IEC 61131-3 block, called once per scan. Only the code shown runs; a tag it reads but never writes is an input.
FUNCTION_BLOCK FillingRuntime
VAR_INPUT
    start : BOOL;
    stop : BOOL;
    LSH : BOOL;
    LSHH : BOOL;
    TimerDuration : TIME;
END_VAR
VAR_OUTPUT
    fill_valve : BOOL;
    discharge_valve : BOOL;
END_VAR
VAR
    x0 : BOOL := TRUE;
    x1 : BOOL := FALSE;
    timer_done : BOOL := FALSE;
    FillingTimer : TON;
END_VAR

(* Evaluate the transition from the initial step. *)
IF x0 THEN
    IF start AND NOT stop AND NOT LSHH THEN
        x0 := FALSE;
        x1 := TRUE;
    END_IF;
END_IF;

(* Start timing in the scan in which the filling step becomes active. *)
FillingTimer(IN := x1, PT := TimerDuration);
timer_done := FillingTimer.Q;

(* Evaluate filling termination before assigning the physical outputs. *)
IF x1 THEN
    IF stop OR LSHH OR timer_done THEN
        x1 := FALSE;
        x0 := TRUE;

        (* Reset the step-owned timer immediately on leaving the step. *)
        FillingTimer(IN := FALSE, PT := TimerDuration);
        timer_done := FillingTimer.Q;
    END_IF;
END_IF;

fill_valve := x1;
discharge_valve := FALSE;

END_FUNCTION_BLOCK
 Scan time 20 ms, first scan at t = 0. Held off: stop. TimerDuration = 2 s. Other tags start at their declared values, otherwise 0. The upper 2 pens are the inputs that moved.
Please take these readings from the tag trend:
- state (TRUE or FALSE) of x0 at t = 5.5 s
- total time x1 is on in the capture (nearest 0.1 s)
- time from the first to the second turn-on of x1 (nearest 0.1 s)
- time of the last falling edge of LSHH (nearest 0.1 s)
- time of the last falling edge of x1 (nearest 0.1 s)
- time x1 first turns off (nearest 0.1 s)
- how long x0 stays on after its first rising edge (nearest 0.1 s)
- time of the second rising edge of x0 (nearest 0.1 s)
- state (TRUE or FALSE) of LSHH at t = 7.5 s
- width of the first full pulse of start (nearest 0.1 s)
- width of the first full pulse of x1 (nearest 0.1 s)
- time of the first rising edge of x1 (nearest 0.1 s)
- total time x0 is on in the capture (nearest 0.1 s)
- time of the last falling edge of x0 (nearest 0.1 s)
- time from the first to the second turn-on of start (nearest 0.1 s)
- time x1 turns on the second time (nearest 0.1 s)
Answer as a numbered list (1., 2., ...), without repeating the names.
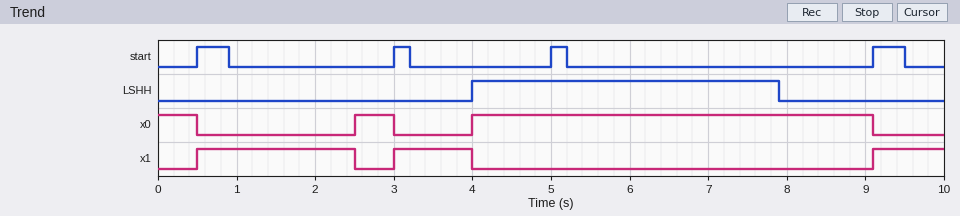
1. TRUE
2. 3.9 s
3. 2.5 s
4. 7.9 s
5. 4.0 s
6. 2.5 s
7. 0.5 s
8. 4.0 s
9. TRUE
10. 0.4 s
11. 2.0 s
12. 0.5 s
13. 6.1 s
14. 9.1 s
15. 2.5 s
16. 3.0 s
